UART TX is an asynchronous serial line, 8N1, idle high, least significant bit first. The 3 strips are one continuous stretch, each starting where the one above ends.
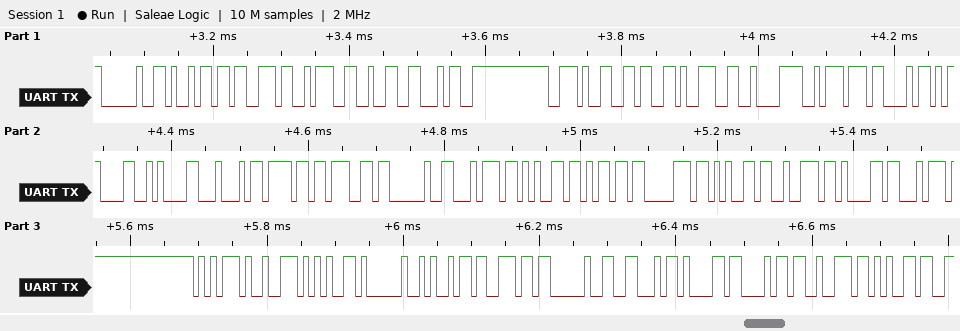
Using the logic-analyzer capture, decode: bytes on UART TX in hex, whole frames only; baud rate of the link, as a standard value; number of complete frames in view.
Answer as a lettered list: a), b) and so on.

a) 20 69 73 3A 32 34 2E 36 39 C2 BA 43 0D 0A 44 6F 67 20 74 65 6D 70 65 72 61 74 75 72 65 20 69 6E 20 46 61 68 72 65
b) 115200 baud
c) 38
